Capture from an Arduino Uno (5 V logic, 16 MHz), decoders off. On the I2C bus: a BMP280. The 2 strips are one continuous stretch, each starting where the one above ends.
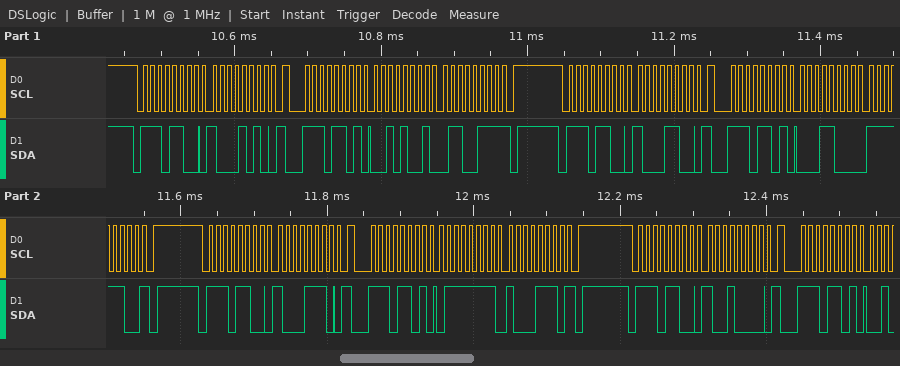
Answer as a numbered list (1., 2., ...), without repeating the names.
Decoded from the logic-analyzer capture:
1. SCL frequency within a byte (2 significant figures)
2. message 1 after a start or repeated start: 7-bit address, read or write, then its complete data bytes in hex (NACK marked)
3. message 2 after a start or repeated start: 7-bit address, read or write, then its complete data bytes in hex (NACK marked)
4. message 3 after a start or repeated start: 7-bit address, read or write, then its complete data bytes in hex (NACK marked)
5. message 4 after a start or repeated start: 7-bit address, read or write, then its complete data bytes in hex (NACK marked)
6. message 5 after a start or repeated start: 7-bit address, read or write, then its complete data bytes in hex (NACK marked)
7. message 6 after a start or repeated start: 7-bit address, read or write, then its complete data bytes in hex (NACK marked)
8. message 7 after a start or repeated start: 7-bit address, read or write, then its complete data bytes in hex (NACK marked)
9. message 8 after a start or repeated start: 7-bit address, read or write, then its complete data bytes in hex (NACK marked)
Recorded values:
1. 100 kHz
2. 0x76 write: 8A
3. 0x76 read: 29 67 NACK
4. 0x76 write: 8C
5. 0x76 read: 18 FC NACK
6. 0x76 write: 8E
7. 0x76 read: 7F 8E NACK
8. 0x76 write: 90
9. 0x76 read
